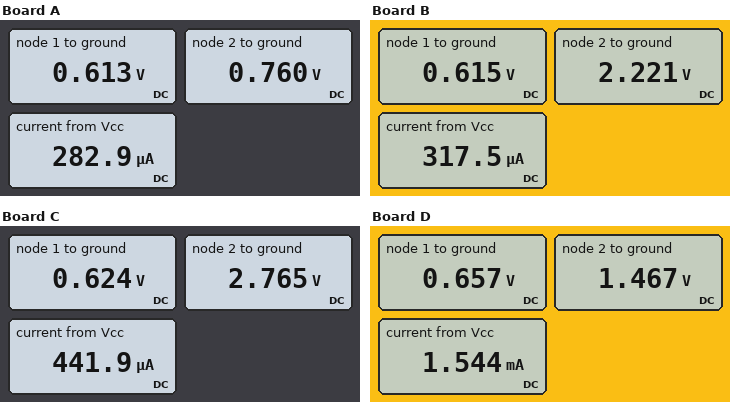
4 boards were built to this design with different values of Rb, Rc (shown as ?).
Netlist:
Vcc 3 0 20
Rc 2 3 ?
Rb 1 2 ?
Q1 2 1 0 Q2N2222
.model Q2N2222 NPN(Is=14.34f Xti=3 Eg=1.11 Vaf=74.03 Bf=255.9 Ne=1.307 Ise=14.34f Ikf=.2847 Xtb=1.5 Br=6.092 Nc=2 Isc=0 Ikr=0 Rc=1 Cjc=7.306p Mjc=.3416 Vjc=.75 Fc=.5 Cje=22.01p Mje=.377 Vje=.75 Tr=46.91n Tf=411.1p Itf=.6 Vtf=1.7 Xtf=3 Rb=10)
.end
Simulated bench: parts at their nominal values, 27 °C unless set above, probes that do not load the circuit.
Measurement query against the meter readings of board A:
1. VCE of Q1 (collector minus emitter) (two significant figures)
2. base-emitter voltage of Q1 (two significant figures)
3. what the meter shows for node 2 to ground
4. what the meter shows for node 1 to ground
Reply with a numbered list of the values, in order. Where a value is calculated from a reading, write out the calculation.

1. 760 mV = 760 mV
2. 613 mV = 610 mV
3. 0.760 V
4. 0.613 V
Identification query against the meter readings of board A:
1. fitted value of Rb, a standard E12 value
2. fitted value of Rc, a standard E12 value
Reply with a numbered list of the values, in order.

1. 68 kΩ
2. 68 kΩ
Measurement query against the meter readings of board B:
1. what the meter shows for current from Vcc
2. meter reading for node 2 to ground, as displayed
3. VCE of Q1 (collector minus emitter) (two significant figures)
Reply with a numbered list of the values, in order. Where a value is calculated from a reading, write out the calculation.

1. 317.5 µA
2. 2.221 V
3. 2.221 V = 2.2 V
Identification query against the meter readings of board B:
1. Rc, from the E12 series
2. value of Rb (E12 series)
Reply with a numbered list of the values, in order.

1. 56 kΩ
2. 680 kΩ
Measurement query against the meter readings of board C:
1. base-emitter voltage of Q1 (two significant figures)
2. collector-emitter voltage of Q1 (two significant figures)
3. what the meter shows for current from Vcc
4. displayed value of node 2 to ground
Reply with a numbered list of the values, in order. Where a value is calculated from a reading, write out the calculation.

1. 624 mV = 620 mV
2. 2.765 V = 2.8 V
3. 441.9 µA
4. 2.765 V
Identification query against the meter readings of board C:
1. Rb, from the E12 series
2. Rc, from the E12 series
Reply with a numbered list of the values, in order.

1. 680 kΩ
2. 39 kΩ
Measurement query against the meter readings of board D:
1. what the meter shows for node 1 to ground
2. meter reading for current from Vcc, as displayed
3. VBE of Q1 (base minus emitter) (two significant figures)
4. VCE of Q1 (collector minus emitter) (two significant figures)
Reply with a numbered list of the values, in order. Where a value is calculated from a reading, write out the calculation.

1. 0.657 V
2. 1.544 mA
3. 657 mV = 660 mV
4. 1.467 V = 1.5 V
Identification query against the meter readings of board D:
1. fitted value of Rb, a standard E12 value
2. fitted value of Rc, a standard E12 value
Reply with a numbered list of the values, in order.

1. 82 kΩ
2. 12 kΩ
